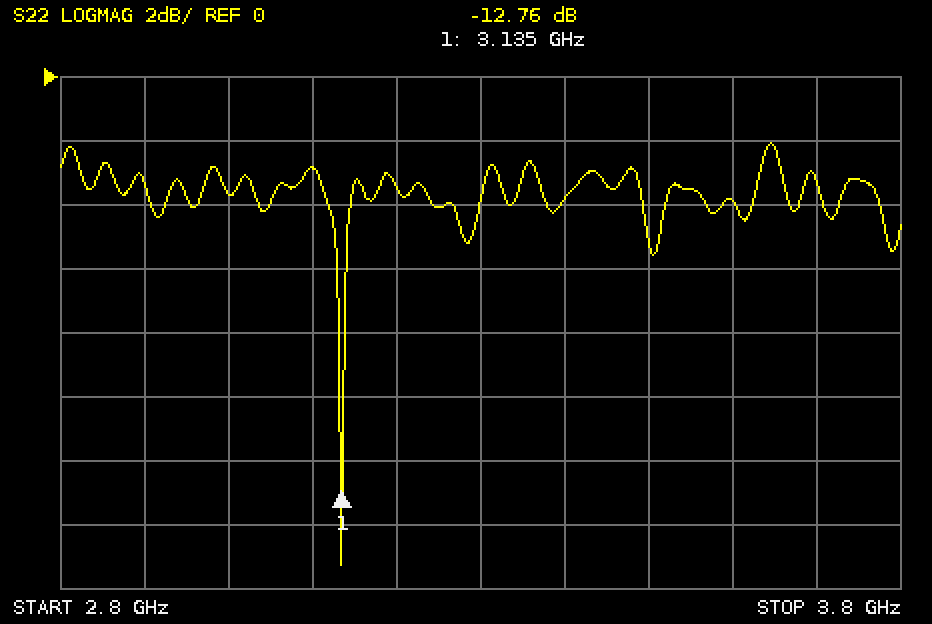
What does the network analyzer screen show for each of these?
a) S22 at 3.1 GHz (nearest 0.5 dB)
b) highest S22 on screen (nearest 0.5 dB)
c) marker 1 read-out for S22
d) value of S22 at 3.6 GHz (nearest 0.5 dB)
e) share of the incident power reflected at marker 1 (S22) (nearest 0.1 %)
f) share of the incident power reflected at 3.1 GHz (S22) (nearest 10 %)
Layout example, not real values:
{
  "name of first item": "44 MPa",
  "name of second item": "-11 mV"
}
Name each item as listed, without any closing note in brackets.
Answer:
{
  "S22 at 3.1 GHz": "-3.0 dB",
  "highest S22 on screen": "-2.0 dB",
  "marker 1 read-out for S22": "-12.76 dB",
  "value of S22 at 3.6 GHz": "-4.0 dB",
  "share of the incident power reflected at marker 1 (S22)": "5.3 %",
  "share of the incident power reflected at 3.1 GHz (S22)": "50 %"
}
